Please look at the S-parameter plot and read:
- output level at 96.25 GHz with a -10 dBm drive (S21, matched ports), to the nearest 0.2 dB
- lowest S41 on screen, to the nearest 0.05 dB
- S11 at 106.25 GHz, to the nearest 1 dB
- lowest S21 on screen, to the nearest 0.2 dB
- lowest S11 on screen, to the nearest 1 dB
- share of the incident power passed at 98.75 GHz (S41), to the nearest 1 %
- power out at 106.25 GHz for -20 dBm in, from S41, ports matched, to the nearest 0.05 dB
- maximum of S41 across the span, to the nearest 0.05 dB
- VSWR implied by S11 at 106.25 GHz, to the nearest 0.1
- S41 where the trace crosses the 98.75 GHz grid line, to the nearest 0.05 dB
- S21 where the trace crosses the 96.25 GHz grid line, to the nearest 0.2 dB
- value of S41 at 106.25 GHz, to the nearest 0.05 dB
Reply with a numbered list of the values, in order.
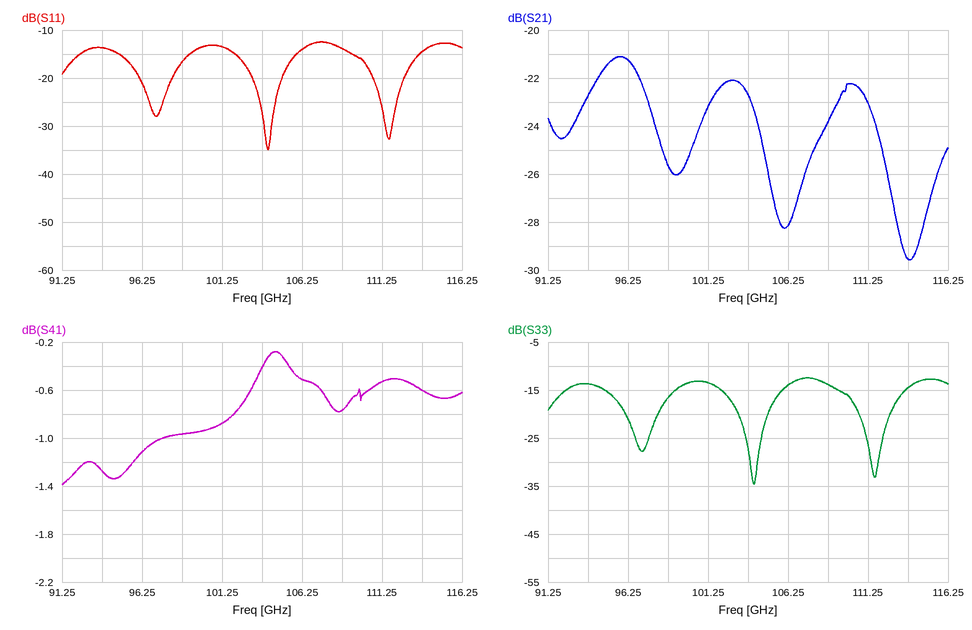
1. -31.2 dBm
2. -1.40 dB
3. -14 dB
4. -29.6 dB
5. -35 dB
6. 80 %
7. -20.50 dBm
8. -0.30 dB
9. 1.5
10. -0.95 dB
11. -21.2 dB
12. -0.50 dB
